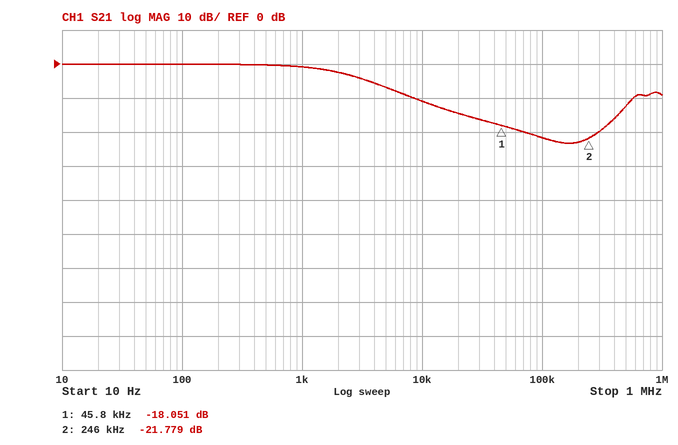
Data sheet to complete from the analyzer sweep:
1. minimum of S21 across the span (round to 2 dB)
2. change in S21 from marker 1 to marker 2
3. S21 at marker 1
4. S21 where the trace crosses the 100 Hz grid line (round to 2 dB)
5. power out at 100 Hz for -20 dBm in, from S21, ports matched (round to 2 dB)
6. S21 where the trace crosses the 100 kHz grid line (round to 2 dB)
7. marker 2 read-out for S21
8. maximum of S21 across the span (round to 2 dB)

-24 dB
-3.728 dB
-18.051 dB
0 dB
-20 dBm
-22 dB
-21.779 dB
0 dB
